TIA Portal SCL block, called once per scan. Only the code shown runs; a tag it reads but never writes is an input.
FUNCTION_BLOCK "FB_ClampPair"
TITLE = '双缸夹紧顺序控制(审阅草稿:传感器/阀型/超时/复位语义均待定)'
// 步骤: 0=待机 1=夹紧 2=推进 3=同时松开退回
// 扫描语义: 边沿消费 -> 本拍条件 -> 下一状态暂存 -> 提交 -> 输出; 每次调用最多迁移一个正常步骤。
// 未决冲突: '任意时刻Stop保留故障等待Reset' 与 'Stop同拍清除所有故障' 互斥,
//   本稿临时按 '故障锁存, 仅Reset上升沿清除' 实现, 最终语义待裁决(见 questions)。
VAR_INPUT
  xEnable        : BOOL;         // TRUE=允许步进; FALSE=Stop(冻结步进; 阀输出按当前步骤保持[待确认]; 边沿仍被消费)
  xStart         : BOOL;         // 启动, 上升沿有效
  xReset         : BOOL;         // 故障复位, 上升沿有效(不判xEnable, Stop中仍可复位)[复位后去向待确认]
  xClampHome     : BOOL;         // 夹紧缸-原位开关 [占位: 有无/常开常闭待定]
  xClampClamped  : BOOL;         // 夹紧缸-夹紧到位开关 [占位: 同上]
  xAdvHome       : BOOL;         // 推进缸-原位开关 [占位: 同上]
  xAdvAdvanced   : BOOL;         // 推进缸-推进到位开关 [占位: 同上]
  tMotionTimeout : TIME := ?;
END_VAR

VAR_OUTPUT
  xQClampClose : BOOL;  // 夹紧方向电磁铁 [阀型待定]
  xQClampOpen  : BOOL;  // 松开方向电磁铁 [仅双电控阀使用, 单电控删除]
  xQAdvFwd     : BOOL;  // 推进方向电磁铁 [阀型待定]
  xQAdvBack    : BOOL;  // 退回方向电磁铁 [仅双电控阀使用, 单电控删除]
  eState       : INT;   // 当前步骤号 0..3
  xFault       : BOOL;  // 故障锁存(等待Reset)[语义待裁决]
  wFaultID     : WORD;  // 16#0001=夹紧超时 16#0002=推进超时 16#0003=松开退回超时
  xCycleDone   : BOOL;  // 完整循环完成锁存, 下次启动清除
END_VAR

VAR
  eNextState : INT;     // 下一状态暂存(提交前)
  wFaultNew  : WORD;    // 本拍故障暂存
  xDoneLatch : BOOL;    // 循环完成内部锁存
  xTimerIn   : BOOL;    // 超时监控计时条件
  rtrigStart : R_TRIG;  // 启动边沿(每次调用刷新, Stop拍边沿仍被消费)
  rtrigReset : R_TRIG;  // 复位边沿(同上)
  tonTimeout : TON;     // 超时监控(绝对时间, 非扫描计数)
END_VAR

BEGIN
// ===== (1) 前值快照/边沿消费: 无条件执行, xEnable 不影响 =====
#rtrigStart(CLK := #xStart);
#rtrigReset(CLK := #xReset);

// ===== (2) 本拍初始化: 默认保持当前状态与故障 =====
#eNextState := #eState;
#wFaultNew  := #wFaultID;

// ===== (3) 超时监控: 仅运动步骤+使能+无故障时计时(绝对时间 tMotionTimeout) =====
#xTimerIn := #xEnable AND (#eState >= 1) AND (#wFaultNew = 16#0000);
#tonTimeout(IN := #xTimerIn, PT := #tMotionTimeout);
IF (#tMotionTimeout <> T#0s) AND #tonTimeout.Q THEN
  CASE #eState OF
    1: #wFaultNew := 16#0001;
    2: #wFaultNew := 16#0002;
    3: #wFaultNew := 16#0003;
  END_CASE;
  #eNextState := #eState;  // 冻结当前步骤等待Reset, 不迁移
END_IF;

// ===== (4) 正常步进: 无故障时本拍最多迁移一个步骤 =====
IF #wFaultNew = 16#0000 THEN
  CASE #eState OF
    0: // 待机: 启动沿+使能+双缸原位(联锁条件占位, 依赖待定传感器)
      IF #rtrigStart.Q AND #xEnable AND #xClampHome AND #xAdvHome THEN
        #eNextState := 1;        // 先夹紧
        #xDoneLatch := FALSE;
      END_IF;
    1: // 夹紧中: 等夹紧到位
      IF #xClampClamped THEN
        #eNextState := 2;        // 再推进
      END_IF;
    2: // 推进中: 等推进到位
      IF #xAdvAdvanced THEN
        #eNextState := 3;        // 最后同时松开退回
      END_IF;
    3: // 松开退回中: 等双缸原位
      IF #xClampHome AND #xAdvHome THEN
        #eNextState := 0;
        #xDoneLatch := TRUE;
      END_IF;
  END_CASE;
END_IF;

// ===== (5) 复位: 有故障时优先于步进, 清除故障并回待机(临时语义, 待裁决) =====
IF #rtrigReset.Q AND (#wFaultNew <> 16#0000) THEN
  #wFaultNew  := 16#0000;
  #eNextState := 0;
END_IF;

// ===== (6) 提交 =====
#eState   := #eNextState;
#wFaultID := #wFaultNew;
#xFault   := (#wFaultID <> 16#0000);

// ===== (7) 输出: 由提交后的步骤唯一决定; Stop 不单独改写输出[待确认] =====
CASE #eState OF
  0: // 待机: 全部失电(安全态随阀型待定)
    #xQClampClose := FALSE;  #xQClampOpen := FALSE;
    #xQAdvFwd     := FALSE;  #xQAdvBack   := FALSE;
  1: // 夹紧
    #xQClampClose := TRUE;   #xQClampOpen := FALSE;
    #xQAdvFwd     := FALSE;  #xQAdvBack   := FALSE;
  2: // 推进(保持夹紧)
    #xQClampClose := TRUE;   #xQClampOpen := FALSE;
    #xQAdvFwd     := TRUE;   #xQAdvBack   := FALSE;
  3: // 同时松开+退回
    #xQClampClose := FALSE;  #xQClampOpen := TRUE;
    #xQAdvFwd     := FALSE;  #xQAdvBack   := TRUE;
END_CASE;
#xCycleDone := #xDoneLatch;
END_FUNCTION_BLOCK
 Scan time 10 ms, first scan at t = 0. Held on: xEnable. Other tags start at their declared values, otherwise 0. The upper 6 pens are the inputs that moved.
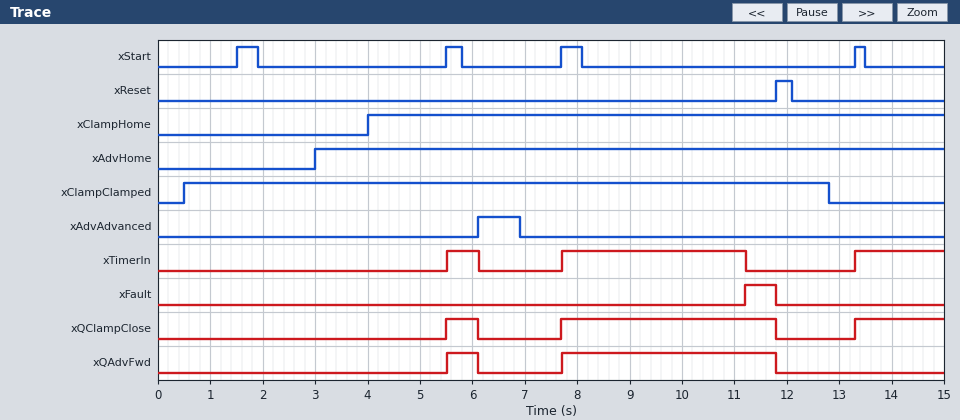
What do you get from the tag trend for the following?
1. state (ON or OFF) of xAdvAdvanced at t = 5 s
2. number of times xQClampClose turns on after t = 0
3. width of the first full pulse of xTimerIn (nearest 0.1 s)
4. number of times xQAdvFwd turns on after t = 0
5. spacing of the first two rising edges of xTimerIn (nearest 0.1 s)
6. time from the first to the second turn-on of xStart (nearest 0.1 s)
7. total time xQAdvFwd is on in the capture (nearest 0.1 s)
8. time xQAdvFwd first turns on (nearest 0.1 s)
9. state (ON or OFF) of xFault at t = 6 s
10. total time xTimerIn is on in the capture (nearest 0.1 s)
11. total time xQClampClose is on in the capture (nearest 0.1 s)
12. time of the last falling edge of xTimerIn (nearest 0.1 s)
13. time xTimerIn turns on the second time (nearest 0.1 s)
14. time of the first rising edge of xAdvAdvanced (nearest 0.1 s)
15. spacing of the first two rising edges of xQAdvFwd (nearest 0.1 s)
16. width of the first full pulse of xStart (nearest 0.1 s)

OFF
3
0.6 s
2
2.2 s
4.0 s
4.7 s
5.5 s
OFF
5.8 s
6.4 s
11.2 s
7.7 s
6.1 s
2.2 s
0.4 s
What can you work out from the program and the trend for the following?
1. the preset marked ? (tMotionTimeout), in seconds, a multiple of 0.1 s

3.5 s
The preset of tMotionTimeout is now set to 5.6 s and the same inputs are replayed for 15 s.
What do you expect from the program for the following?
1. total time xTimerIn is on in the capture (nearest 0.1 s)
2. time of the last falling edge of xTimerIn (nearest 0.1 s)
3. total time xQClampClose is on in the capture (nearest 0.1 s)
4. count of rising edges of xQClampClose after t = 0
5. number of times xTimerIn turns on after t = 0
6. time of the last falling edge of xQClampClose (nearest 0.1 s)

6.2 s
13.3 s
7.9 s
2
2
6.1 s
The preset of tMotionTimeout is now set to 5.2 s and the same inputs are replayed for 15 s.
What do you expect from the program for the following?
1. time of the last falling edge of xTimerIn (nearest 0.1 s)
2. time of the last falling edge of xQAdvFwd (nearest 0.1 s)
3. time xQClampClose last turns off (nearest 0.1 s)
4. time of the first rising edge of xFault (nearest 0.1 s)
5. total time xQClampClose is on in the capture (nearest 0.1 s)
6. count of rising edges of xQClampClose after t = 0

12.9 s
6.1 s
6.1 s
12.9 s
7.9 s
2
